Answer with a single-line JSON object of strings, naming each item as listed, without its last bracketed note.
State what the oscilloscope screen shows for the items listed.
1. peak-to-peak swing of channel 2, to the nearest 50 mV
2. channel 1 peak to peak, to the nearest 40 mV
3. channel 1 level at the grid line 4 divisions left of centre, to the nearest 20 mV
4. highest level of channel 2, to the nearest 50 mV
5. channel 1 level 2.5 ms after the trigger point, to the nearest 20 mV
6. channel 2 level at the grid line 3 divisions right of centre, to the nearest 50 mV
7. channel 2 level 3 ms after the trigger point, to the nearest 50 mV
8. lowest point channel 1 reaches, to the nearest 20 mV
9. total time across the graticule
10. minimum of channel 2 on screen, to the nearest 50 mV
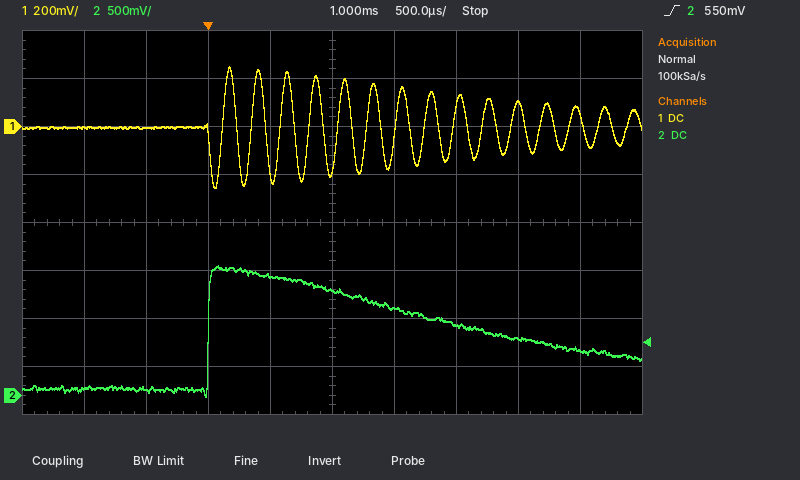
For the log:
{"peak-to-peak swing of channel 2, to the nearest 50 mV": "1.35 V", "channel 1 peak to peak, to the nearest 40 mV": "520 mV", "channel 1 level at the grid line 4 divisions left of centre, to the nearest 20 mV": "0 mV", "highest level of channel 2, to the nearest 50 mV": "1.35 V", "channel 1 level 2.5 ms after the trigger point, to the nearest 20 mV": "100 mV", "channel 2 level at the grid line 3 divisions right of centre, to the nearest 50 mV": "600 mV", "channel 2 level 3 ms after the trigger point, to the nearest 50 mV": "450 mV", "lowest point channel 1 reaches, to the nearest 20 mV": "-260 mV", "total time across the graticule": "5 ms", "minimum of channel 2 on screen, to the nearest 50 mV": "0 mV"}
